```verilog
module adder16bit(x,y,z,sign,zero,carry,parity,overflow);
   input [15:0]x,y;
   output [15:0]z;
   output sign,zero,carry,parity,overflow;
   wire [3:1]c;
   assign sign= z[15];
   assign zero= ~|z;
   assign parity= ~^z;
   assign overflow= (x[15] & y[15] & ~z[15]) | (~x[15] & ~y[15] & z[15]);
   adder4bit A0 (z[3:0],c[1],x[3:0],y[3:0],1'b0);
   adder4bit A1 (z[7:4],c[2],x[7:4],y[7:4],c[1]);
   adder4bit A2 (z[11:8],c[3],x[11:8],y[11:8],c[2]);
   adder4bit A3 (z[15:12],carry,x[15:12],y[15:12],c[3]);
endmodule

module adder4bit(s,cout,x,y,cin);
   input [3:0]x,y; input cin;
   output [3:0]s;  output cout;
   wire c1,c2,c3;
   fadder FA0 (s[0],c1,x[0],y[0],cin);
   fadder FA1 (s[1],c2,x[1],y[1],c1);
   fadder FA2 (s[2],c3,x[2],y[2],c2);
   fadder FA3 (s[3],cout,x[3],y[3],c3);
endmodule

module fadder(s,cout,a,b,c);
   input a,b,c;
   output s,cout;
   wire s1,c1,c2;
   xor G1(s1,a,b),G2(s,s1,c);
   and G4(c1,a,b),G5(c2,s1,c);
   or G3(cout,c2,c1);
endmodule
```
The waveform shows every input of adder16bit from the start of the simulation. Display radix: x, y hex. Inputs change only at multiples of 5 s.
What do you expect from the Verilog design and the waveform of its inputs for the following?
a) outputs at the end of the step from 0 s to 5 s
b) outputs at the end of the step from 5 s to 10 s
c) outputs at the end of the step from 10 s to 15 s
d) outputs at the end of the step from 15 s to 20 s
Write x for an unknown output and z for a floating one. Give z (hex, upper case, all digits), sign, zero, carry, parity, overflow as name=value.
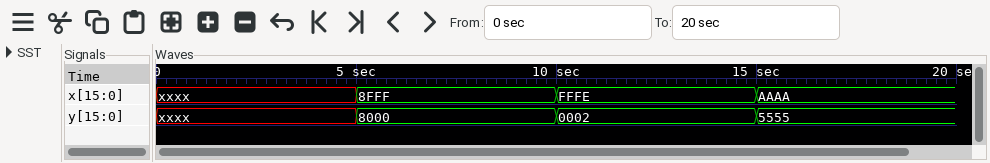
z=x, sign=x, zero=x, carry=x, parity=x, overflow=x
z=0FFF, sign=0, zero=0, carry=1, parity=1, overflow=1
z=0000, sign=0, zero=1, carry=1, parity=1, overflow=0
z=FFFF, sign=1, zero=0, carry=0, parity=1, overflow=0
